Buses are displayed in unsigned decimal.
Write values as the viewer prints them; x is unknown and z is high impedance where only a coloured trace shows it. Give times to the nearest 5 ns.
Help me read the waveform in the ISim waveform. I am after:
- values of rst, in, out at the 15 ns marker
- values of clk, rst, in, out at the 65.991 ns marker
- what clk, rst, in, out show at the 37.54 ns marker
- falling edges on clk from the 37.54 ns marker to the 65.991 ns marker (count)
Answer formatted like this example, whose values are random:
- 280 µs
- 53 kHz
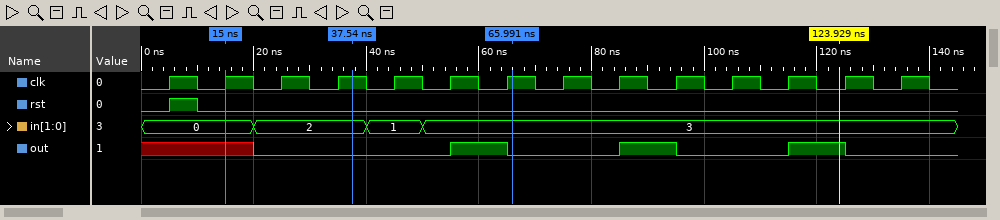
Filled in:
- rst=0, in=0, out=x
- clk=1, rst=0, in=3, out=0
- clk=1, rst=0, in=2, out=0
- 3
